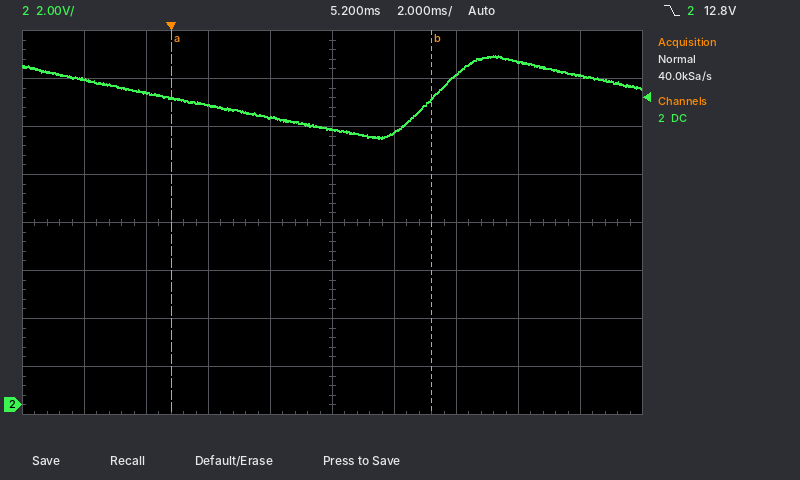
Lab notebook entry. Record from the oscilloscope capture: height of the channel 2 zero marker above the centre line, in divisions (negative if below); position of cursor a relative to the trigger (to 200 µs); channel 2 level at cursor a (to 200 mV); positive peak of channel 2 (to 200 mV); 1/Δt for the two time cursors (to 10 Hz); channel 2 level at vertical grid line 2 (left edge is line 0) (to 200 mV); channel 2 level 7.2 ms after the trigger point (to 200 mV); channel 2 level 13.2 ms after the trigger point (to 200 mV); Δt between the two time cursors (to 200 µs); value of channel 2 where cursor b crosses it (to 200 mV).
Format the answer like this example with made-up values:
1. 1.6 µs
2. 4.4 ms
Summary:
1. -3.8 div
2. 0.0 ms
3. 12.8 V
4. 14.6 V
5. 120 Hz
6. 13.0 V
7. 11.4 V
8. 13.8 V
9. 8.4 ms
10. 12.8 V
